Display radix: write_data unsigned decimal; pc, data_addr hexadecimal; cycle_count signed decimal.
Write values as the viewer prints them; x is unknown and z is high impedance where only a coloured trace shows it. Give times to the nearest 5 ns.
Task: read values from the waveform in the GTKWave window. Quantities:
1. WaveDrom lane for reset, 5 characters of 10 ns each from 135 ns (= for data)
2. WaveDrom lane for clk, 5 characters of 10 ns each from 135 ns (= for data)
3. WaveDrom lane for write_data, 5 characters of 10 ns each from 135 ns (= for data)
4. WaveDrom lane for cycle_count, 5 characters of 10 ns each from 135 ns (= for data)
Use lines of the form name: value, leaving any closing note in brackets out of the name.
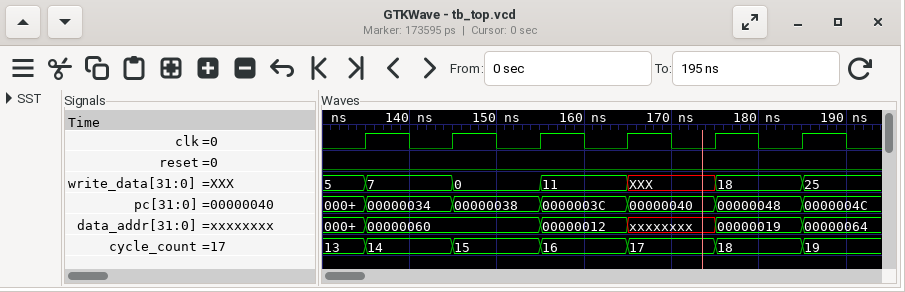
WaveDrom lane for reset, 5 characters of 10 ns each from 135 ns: {name: 'reset', wave: '0....'}
WaveDrom lane for clk, 5 characters of 10 ns each from 135 ns: {name: 'clk', wave: 'p....'}
WaveDrom lane for write_data, 5 characters of 10 ns each from 135 ns: {name: 'write_data', wave: '===x=', data: '7 0 11 18'}
WaveDrom lane for cycle_count, 5 characters of 10 ns each from 135 ns: {name: 'cycle_count', wave: '=====', data: '14 15 16 17 18'}
